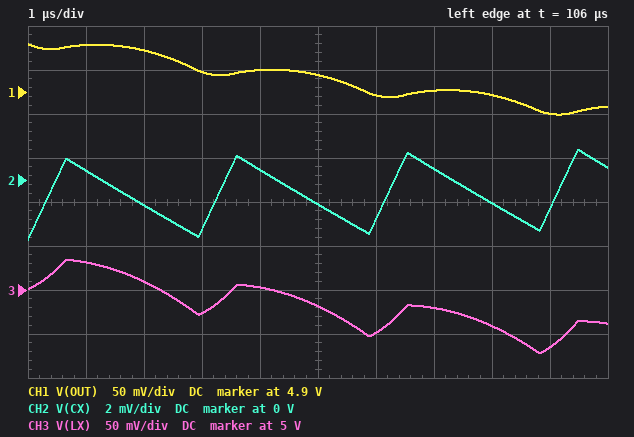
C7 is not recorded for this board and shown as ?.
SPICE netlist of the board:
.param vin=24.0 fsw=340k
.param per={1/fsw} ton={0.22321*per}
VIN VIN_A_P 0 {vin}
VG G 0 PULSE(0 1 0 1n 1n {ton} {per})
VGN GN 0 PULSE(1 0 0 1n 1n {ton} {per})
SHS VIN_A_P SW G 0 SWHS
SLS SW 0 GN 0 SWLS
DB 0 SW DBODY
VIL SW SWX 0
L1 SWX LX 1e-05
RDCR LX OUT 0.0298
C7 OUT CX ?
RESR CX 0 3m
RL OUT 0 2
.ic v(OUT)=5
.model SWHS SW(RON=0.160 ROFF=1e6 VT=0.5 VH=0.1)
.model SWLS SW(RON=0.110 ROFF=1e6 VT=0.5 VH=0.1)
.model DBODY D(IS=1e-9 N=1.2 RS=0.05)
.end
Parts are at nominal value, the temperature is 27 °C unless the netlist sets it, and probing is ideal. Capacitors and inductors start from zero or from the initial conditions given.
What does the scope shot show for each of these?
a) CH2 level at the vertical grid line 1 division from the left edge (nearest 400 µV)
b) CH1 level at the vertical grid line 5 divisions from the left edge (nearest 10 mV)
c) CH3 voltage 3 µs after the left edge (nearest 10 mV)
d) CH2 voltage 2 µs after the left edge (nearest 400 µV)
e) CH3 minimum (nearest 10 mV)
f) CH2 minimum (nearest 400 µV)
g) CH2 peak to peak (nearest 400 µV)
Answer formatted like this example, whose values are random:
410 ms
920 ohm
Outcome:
400 µV
4.92 V
4.97 V
-1.2 mV
4.93 V
-2.8 mV
4.0 mV
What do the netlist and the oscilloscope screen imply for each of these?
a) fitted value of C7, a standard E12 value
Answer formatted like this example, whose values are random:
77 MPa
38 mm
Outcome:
27 µF
